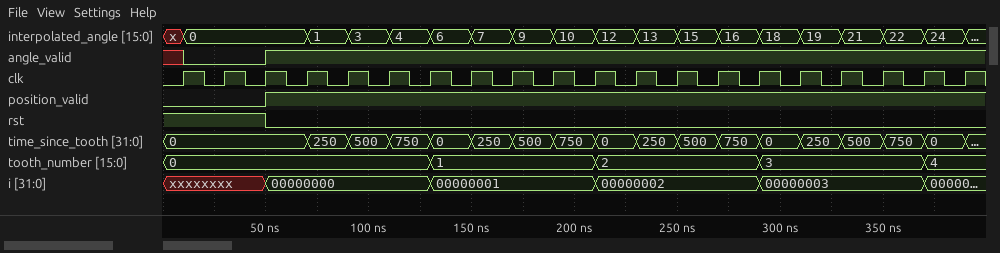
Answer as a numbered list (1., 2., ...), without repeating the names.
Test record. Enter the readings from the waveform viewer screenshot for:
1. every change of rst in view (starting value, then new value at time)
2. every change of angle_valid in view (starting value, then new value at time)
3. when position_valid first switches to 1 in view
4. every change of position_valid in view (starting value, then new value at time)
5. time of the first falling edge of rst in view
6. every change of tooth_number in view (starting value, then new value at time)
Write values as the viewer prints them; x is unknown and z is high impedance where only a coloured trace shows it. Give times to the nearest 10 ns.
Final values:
1. 1, 0 at 50 ns
2. x, 0 at 10 ns, 1 at 50 ns
3. 50 ns
4. 0, 1 at 50 ns
5. 50 ns
6. 0, 1 at 130 ns, 2 at 210 ns, 3 at 290 ns, 4 at 370 ns
